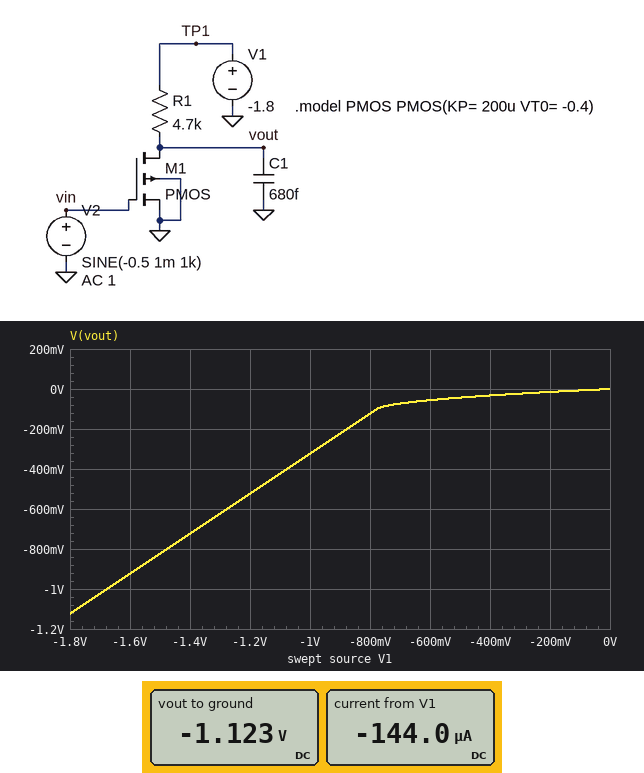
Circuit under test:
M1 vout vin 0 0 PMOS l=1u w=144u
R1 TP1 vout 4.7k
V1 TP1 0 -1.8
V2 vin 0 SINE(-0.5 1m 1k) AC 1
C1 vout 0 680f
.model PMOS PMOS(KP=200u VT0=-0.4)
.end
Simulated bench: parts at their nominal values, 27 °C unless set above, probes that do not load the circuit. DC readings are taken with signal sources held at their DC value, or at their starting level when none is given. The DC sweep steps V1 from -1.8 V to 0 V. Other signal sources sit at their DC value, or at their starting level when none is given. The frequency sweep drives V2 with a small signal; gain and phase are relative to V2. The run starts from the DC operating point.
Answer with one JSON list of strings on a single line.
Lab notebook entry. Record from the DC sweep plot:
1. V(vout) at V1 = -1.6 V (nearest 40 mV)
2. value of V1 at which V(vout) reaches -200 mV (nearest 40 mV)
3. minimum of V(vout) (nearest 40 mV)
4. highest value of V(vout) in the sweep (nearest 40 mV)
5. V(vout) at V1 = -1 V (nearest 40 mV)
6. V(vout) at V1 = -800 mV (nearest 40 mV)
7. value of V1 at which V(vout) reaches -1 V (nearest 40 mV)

["-920 mV", "-880 mV", "-1.12 V", "0 V", "-320 mV", "-120 mV", "-1.68 V"]
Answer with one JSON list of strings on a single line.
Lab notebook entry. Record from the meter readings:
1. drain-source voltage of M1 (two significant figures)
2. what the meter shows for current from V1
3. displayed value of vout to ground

["-1.1 V", "-144.0 µA", "-1.123 V"]
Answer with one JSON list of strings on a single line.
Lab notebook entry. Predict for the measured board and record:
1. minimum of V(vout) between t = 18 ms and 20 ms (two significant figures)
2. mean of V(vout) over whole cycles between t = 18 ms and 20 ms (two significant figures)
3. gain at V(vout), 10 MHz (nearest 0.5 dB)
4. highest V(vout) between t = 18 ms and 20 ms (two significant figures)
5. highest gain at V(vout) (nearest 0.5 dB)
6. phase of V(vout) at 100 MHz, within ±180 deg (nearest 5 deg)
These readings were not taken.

["-1.1 V", "-1.1 V", "22.5 dB", "-1.1 V", "22.5 dB", "115 deg"]
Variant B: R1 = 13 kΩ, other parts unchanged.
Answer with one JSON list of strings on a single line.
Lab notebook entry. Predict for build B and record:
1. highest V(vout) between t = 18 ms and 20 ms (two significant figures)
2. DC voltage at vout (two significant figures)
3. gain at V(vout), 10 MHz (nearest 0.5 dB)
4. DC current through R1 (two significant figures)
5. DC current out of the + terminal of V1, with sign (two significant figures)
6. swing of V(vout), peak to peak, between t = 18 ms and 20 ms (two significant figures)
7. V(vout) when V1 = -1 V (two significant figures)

["-70 mV", "-72 mV", "7.5 dB", "130 µA", "-130 µA", "4.8 mV", "-31 mV"]
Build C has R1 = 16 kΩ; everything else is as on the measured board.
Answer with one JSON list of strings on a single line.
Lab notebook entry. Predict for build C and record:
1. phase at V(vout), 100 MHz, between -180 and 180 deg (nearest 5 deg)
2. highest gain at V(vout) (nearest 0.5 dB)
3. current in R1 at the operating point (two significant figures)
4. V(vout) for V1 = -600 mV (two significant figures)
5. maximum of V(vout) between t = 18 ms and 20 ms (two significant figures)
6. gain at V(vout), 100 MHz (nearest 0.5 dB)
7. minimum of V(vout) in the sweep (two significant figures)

["165 deg", "0 dB", "110 µA", "-14 mV", "-50 mV", "-0.5 dB", "-51 mV"]
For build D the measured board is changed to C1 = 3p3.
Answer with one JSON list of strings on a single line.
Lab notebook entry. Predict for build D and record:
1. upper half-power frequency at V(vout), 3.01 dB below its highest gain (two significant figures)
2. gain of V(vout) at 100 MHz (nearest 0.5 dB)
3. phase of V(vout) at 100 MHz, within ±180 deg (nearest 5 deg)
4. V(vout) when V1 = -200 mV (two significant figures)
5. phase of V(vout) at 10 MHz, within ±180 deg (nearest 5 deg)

["10 MHz", "3.0 dB", "95 deg", "-15 mV", "135 deg"]
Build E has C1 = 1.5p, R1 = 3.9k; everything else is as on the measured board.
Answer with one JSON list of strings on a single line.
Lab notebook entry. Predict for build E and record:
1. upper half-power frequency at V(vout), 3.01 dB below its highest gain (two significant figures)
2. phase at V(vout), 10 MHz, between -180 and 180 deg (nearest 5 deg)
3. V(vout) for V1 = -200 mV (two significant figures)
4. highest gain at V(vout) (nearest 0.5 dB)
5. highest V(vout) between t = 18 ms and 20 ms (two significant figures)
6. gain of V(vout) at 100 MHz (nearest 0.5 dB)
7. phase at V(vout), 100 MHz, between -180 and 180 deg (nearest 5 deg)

["27 MHz", "160 deg", "-18 mV", "21.0 dB", "-1.2 V", "9.5 dB", "105 deg"]
